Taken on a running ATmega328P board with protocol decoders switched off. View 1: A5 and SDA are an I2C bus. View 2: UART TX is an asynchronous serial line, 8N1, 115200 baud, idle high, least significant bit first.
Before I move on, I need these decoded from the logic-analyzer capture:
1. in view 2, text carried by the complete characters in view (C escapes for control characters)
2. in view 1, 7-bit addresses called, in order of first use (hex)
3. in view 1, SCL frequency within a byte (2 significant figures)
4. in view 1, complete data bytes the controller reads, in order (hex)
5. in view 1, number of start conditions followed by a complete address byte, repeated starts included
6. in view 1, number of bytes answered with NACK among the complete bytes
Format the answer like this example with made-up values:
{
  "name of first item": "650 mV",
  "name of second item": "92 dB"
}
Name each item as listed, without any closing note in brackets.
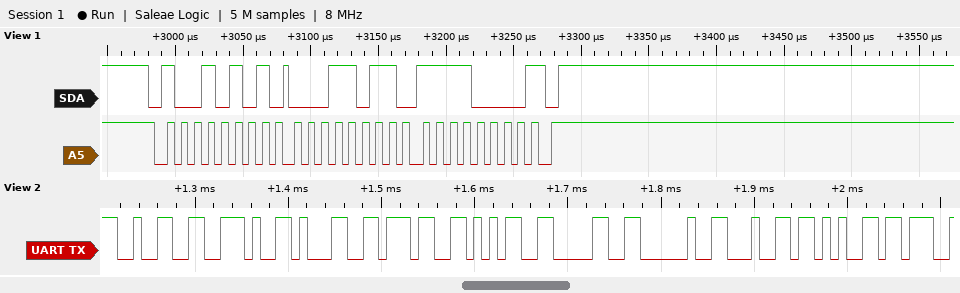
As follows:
{
  "in view 2, text carried by the complete characters in view": "\"2.1750 de\"",
  "in view 1, 7-bit addresses called, in order of first use": "0x4A",
  "in view 1, SCL frequency within a byte": "100 kHz",
  "in view 1, complete data bytes the controller reads, in order": "1B F0",
  "in view 1, number of start conditions followed by a complete address byte, repeated starts included": "1",
  "in view 1, number of bytes answered with NACK among the complete bytes": "1"
}
